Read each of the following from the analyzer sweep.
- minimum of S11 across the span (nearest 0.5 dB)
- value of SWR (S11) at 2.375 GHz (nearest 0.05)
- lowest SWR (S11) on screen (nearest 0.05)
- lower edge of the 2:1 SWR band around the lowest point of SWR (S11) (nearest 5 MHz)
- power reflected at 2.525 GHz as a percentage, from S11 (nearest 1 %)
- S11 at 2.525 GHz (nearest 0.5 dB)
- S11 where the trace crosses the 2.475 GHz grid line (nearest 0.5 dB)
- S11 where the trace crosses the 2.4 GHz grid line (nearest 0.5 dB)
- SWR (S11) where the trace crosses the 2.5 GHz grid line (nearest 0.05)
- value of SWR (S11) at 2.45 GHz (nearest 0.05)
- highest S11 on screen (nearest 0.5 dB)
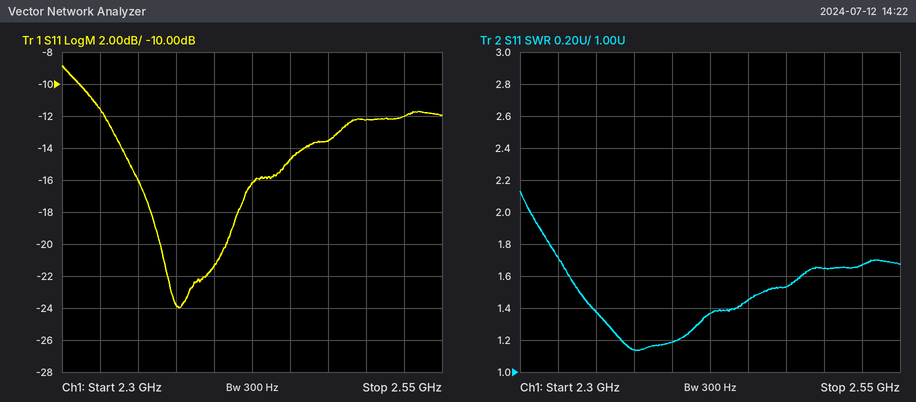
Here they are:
-24.0 dB
1.15
1.15
2.305 GHz
6 %
-12.0 dB
-13.5 dB
-21.5 dB
1.65
1.45
-9.0 dB
